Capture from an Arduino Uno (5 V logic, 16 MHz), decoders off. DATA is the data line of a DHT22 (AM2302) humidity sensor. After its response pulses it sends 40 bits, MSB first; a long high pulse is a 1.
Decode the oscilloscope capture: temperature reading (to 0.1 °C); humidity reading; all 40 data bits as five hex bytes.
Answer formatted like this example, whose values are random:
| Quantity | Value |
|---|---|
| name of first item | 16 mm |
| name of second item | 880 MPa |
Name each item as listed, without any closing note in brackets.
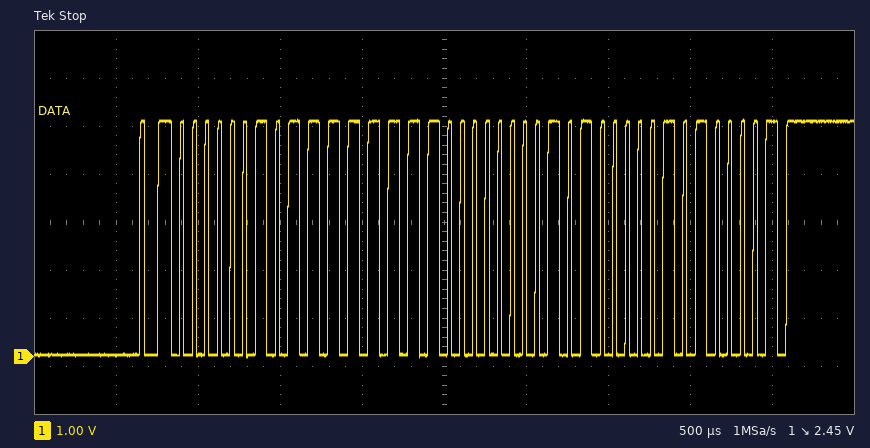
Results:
| Quantity | Value |
|---|---|
| temperature reading | 16.0 °C |
| humidity reading | 76.7 % |
| all 40 data bits as five hex bytes | 02 FF 00 A0 A1 |
